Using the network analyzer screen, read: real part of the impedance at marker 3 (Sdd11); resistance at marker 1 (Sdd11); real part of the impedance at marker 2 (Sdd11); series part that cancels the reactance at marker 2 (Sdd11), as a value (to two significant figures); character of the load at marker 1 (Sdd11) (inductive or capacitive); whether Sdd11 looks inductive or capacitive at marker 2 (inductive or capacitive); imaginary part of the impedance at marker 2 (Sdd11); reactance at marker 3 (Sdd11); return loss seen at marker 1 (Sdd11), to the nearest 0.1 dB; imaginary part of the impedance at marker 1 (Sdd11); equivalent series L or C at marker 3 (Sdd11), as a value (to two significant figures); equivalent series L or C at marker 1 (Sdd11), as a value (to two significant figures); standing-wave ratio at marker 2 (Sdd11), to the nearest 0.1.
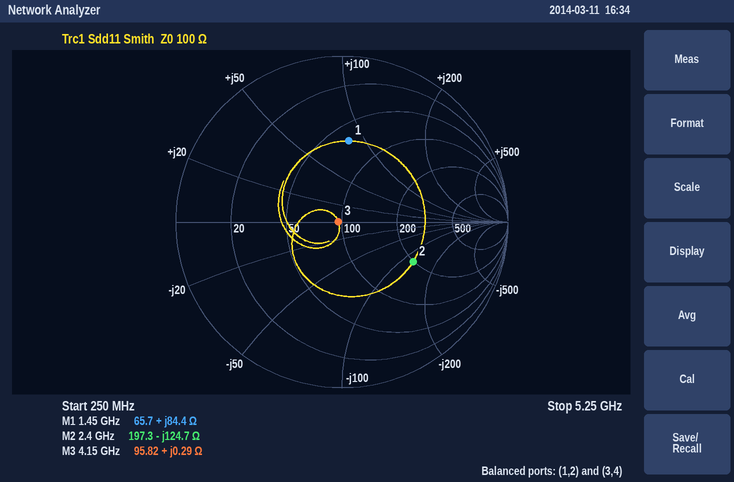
95.82 Ω
65.7 Ω
197.3 Ω
8.3 nH
inductive
capacitive
-124.7 Ω
+0.29 Ω
6.2 dB
+84.4 Ω
11 pH
9.3 nH
2.9
